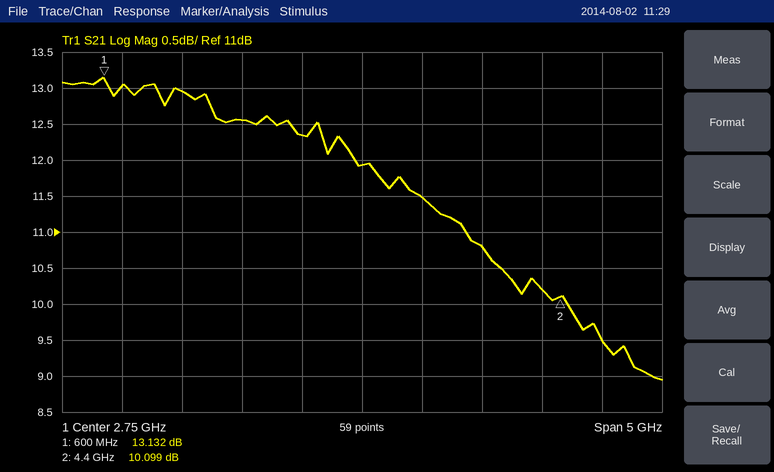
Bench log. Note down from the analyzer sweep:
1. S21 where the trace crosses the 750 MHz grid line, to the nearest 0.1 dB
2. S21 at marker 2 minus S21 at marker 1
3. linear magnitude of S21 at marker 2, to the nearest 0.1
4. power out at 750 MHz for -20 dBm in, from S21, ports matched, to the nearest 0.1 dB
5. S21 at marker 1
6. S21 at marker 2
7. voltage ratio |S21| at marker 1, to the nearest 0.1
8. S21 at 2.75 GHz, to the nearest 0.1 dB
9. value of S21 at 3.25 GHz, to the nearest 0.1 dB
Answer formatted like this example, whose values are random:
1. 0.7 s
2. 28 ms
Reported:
1. 13.0 dB
2. -3.033 dB
3. 3.2
4. -7.0 dBm
5. 13.132 dB
6. 10.099 dB
7. 4.5
8. 11.9 dB
9. 11.5 dB
